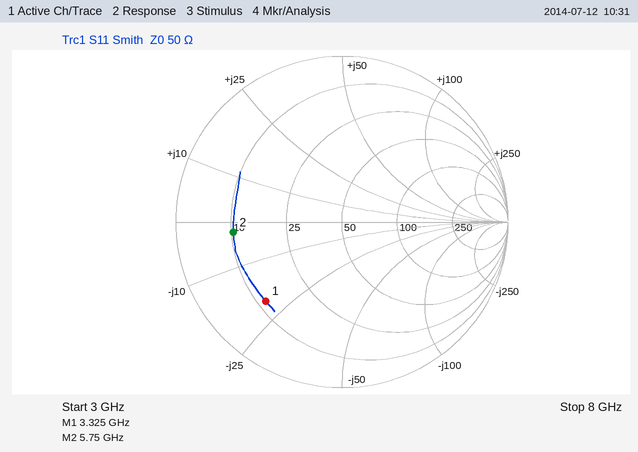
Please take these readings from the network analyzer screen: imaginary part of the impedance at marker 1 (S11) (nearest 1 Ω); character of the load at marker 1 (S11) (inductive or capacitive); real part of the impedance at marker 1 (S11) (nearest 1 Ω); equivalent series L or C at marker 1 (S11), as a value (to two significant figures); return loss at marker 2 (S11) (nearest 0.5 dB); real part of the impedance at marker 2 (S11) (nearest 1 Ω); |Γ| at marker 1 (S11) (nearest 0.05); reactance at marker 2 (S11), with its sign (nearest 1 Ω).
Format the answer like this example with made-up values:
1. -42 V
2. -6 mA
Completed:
1. -20 Ω
2. capacitive
3. 12 Ω
4. 2.4 pF
5. 3.5 dB
6. 10 Ω
7. 0.65
8. -2 Ω
